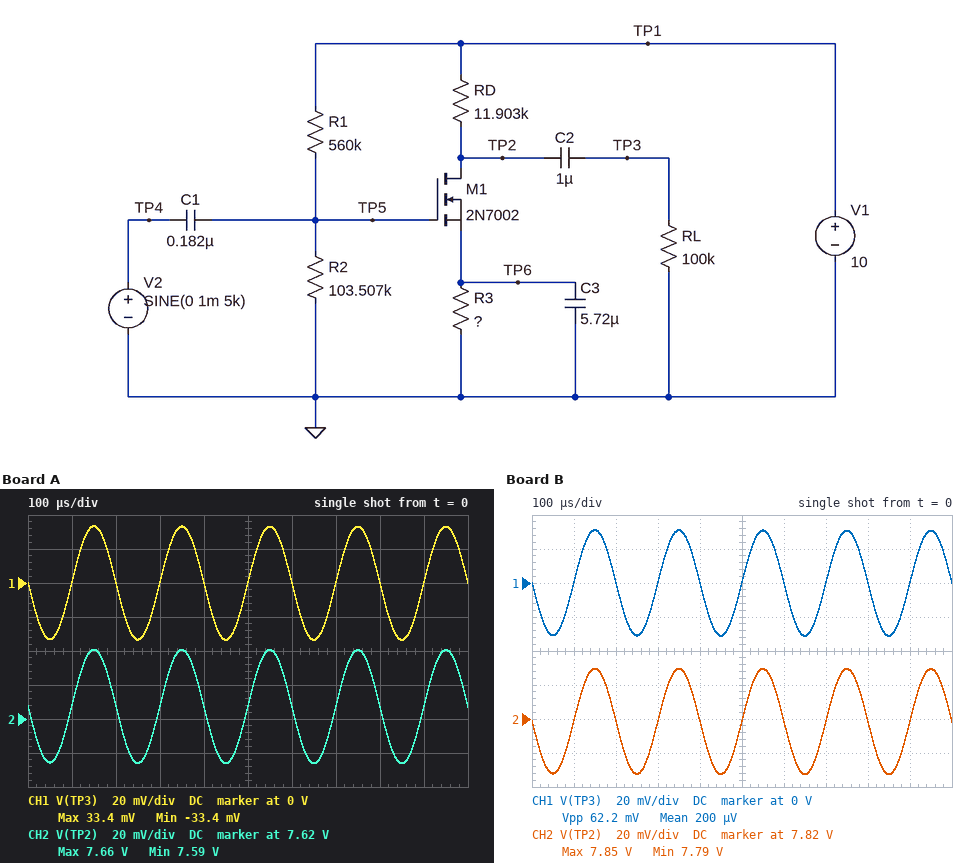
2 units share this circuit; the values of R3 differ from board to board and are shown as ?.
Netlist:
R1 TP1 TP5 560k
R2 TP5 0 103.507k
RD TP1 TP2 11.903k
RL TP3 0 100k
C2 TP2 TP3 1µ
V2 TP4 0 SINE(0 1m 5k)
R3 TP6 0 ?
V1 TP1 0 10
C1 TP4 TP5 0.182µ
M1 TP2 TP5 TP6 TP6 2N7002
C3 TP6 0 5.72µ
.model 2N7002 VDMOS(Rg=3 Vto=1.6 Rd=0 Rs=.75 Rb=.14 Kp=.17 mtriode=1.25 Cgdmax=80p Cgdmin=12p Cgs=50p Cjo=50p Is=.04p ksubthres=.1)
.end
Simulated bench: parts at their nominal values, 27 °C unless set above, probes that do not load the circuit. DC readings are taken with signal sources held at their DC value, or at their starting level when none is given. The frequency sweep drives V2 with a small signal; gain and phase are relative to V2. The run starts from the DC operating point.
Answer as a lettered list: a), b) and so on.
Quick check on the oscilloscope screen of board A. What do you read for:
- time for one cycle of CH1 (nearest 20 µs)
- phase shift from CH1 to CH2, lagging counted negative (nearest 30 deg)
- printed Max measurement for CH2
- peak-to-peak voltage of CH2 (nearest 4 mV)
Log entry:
a) 200 µs
b) 0 deg
c) 7.66 V
d) 68 mV
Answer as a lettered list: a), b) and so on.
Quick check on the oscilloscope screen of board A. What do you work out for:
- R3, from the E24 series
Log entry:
a) 36 Ω
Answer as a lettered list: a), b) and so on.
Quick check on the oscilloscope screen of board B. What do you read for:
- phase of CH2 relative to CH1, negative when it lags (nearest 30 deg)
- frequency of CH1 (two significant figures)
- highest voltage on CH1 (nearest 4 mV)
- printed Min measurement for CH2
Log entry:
a) 0 deg
b) 5.0 kHz
c) 32 mV
d) 7.79 V
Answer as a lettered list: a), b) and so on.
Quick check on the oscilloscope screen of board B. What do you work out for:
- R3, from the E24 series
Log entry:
a) 68 Ω
